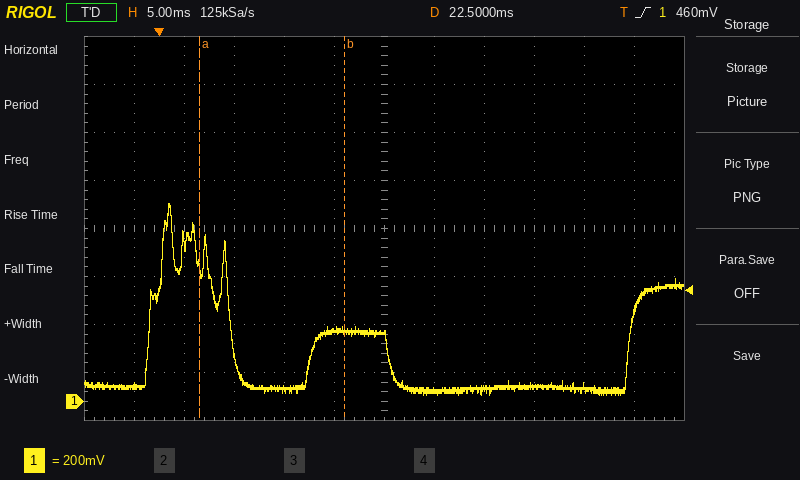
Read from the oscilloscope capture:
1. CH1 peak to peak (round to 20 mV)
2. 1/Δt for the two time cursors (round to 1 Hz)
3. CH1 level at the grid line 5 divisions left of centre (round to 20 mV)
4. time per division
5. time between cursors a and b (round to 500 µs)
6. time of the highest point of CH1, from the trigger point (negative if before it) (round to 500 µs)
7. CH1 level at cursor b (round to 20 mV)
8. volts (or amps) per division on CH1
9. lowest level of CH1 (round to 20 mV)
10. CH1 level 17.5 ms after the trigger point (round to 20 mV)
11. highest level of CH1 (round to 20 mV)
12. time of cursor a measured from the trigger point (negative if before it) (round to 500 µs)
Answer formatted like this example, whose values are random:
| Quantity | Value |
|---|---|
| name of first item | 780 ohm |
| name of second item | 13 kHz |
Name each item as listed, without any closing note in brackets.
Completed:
| Quantity | Value |
|---|---|
| CH1 peak to peak | 800 mV |
| 1/Δt for the two time cursors | 69 Hz |
| CH1 level at the grid line 5 divisions left of centre | 60 mV |
| time per division | 5 ms |
| time between cursors a and b | 14.5 ms |
| time of the highest point of CH1, from the trigger point (negative if before it) | +1.0 ms |
| CH1 level at cursor b | 300 mV |
| volts (or amps) per division on CH1 | 200 mV |
| lowest level of CH1 | 20 mV |
| CH1 level 17.5 ms after the trigger point | 300 mV |
| highest level of CH1 | 820 mV |
| time of cursor a measured from the trigger point (negative if before it) | +4.0 ms |
